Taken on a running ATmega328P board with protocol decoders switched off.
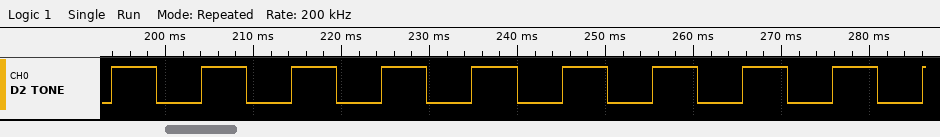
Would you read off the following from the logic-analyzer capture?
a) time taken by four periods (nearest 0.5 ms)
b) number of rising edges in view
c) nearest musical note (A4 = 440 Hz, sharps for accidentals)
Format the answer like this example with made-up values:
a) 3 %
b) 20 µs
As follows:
a) 41.0 ms
b) 10
c) G2
